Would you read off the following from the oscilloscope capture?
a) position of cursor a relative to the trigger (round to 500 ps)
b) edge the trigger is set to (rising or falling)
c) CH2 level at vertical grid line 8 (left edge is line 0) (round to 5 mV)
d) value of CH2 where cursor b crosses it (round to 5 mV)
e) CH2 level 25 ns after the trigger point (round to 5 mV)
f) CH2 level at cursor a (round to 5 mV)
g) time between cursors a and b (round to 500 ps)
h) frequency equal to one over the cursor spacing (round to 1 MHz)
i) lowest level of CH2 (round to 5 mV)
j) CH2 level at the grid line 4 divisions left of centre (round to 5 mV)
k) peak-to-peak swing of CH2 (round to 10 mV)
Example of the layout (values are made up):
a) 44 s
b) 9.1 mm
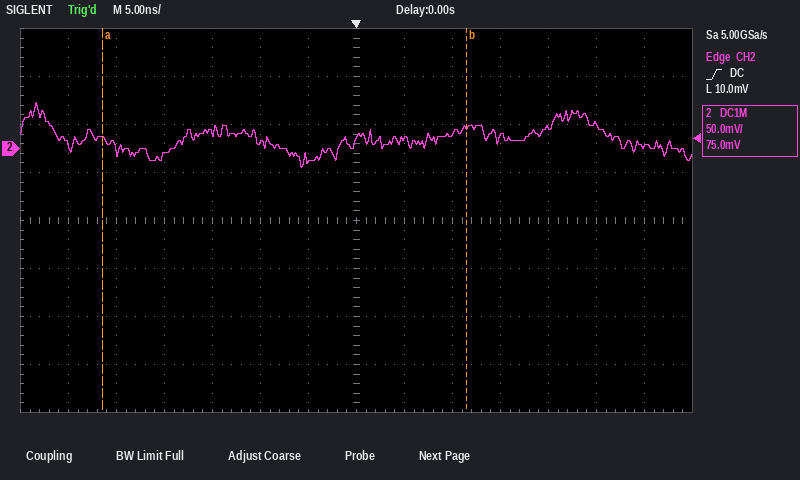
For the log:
a) -26.5 ns
b) rising
c) 10 mV
d) 20 mV
e) 25 mV
f) 10 mV
g) 38.0 ns
h) 26 MHz
i) -20 mV
j) -5 mV
k) 70 mV
